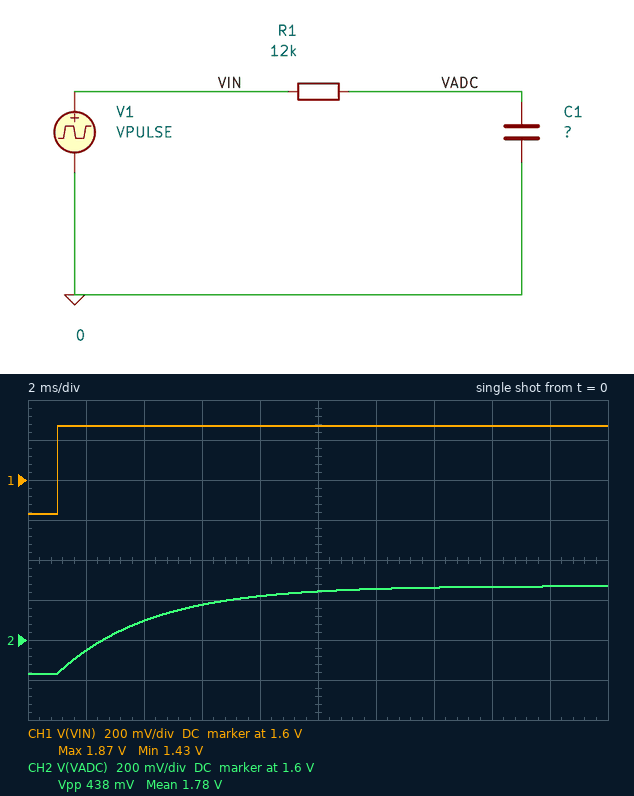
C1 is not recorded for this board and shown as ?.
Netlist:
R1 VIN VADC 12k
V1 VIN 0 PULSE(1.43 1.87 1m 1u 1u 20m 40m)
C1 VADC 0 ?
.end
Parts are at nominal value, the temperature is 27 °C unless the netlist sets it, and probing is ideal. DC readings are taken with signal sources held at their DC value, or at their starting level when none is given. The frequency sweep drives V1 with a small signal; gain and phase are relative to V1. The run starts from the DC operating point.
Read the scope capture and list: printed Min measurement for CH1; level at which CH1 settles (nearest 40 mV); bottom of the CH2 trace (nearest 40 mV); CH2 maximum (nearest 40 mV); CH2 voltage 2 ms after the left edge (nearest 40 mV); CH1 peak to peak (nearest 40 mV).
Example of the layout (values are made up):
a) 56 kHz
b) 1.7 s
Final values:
a) 1.43 V
b) 1.88 V
c) 1.44 V
d) 1.88 V
e) 1.56 V
f) 440 mV
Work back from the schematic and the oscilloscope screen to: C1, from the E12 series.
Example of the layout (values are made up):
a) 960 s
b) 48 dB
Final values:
a) 270 nF
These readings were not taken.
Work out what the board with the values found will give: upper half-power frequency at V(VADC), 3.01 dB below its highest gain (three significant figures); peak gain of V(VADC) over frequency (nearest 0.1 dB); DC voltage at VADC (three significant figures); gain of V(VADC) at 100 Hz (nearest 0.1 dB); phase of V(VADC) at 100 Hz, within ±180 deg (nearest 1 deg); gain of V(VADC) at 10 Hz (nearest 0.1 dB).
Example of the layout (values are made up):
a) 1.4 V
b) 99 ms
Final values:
a) 49.1 Hz
b) 0 dB
c) 1.43 V
d) -7.1 dB
e) -64 deg
f) -0.2 dB
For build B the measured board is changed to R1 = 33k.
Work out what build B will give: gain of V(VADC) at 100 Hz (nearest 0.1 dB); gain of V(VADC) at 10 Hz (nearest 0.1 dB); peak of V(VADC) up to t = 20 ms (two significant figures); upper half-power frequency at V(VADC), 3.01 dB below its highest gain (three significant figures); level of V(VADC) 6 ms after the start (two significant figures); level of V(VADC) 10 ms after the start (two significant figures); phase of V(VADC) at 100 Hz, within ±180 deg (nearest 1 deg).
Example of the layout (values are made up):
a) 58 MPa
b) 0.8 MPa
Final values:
a) -15.1 dB
b) -1.2 dB
c) 1.8 V
d) 17.9 Hz
e) 1.6 V
f) 1.7 V
g) -80 deg
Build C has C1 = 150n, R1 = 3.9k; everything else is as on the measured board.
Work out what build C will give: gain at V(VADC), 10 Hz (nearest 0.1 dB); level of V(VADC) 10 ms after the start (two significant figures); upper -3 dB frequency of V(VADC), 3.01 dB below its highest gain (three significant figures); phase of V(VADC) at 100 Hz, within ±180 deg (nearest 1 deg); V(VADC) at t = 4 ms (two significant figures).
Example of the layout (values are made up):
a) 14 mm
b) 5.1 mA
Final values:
a) 0 dB
b) 1.9 V
c) 272 Hz
d) -20 deg
e) 1.9 V
